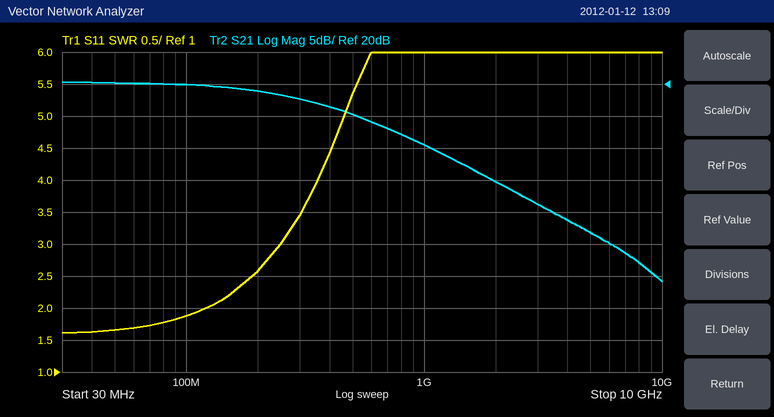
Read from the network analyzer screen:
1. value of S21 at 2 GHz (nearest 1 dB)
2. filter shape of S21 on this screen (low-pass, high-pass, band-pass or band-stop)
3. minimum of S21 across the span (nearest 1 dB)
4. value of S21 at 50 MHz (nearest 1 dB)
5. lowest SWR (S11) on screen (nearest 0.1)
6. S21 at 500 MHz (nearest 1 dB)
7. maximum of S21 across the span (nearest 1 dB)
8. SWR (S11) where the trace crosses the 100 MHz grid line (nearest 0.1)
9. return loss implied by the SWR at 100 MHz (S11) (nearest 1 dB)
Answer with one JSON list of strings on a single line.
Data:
["5 dB", "low-pass", "-11 dB", "20 dB", "1.6", "15 dB", "20 dB", "1.9", "10 dB"]
